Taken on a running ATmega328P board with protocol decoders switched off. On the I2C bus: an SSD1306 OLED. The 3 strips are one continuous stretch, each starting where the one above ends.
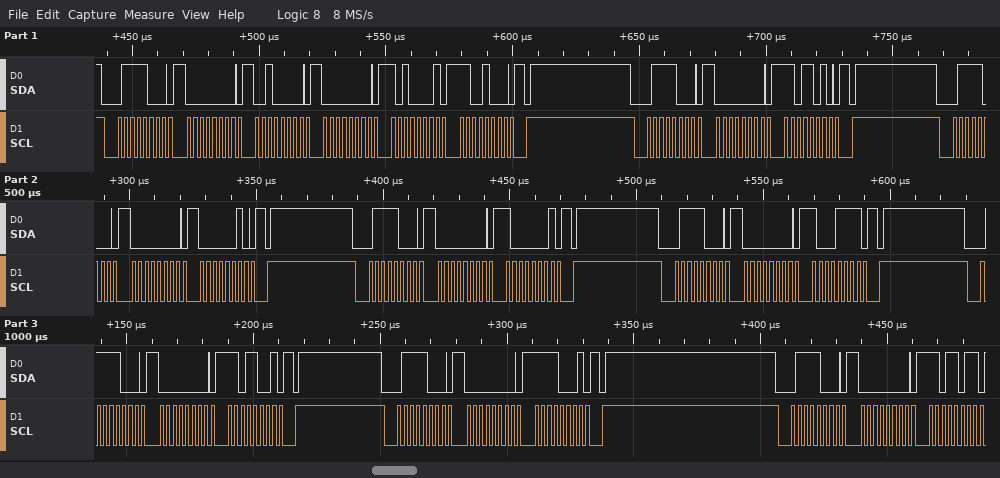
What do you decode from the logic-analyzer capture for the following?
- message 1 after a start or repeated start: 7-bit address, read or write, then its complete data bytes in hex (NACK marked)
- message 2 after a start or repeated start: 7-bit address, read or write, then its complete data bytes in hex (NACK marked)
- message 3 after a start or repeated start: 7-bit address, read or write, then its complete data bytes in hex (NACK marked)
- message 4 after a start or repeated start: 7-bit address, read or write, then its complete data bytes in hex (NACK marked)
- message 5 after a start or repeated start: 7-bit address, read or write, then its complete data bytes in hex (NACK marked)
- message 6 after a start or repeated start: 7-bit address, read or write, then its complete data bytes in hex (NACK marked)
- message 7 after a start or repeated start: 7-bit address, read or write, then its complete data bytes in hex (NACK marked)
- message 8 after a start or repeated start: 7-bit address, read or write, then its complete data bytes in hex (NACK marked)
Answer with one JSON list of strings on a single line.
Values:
["0x3C write: 00 20 00 A1 C8", "0x3C write: 00 DA", "0x3C write: 00 02", "0x3C write: 00 81", "0x3C write: 00 8F", "0x3C write: 00 D9", "0x3C write: 00 F1", "0x3C write: 00 DB"]
